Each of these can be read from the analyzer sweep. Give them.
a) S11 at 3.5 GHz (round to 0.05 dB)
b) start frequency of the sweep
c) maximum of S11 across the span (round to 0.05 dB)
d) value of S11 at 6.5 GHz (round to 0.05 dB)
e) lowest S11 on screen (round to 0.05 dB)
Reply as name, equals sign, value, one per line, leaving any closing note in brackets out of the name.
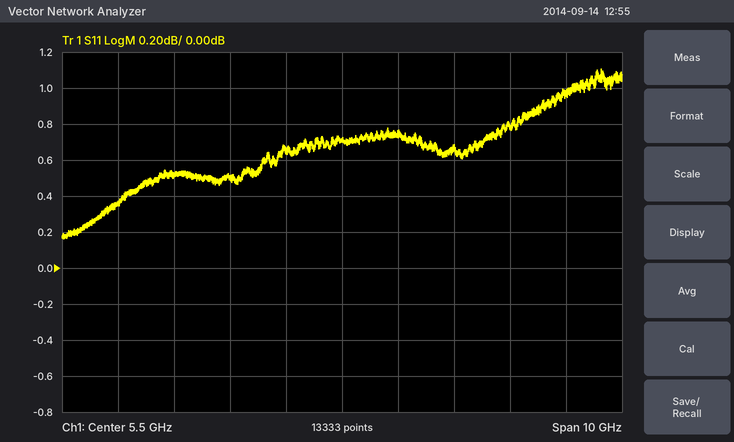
S11 at 3.5 GHz = 0.50 dB
start frequency of the sweep = 500 MHz
maximum of S11 across the span = 1.10 dB
value of S11 at 6.5 GHz = 0.75 dB
lowest S11 on screen = 0.15 dB
